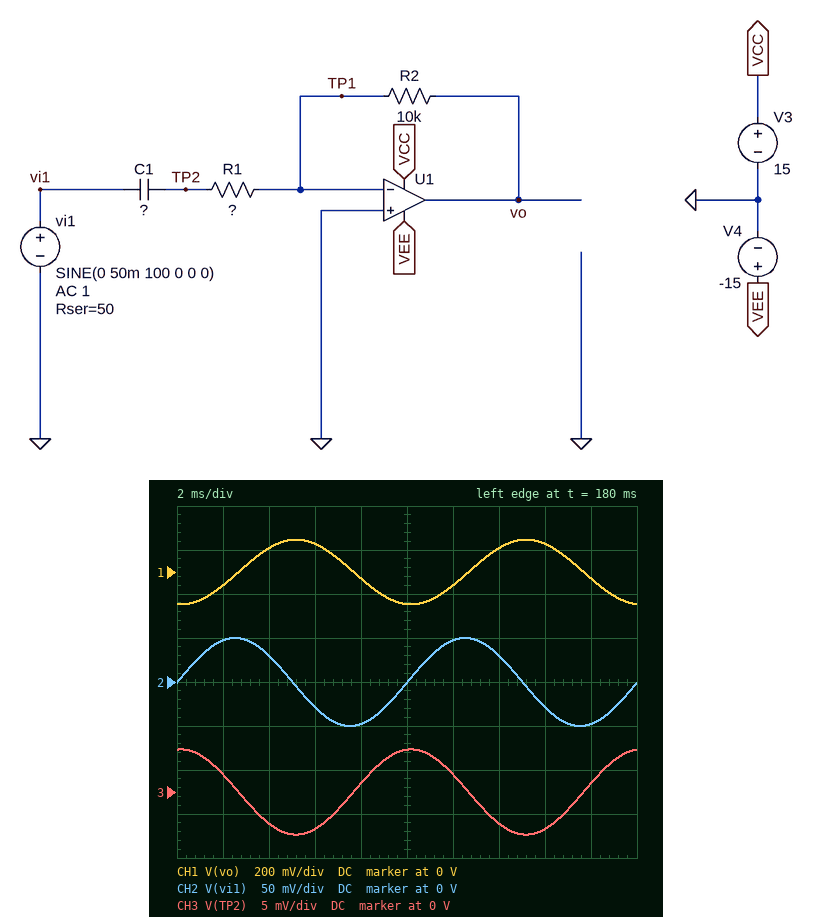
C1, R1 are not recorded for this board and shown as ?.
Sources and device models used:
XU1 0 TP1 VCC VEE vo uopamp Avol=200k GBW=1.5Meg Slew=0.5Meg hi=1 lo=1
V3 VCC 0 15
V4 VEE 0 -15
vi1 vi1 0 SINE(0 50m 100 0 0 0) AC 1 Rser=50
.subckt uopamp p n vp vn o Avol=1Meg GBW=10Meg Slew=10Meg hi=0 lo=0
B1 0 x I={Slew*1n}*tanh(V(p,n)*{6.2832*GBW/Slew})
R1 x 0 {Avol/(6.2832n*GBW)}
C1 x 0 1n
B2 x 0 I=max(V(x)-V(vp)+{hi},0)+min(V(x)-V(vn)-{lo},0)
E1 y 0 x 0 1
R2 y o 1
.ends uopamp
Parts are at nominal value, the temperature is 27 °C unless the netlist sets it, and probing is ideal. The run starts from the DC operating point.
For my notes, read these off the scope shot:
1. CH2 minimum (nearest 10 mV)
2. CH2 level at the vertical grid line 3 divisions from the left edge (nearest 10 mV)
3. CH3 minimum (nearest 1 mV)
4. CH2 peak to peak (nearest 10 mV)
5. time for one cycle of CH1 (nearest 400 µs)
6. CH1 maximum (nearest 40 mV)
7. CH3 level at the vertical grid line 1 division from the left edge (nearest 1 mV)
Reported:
-50 mV
-30 mV
-5 mV
100 mV
10.0 ms
160 mV
2 mV
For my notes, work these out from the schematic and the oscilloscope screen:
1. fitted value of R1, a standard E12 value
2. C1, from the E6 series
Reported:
330 Ω
470 nF
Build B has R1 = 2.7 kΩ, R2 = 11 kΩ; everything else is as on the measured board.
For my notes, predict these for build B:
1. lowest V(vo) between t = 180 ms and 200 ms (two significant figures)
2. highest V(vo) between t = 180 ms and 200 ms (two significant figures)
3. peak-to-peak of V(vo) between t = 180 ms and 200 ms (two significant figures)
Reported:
-130 mV
130 mV
250 mV
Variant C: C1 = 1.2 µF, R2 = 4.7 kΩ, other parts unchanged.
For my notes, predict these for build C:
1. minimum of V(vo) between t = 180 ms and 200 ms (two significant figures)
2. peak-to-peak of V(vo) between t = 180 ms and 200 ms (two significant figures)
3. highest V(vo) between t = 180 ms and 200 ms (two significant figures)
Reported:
-170 mV
340 mV
170 mV
